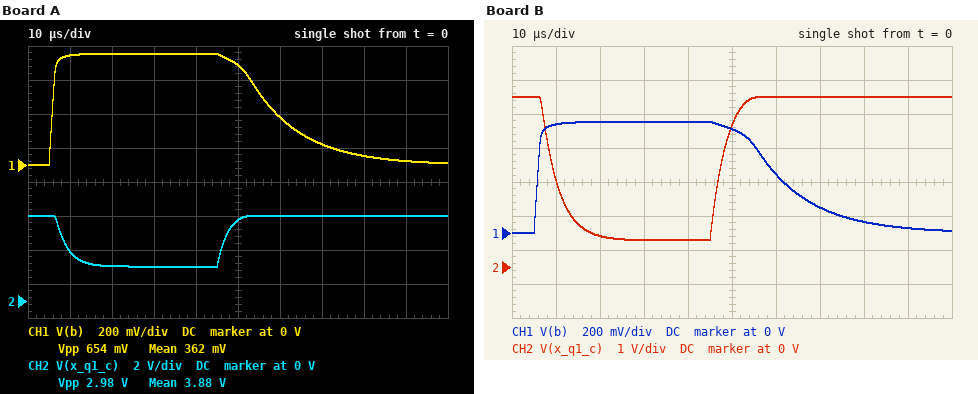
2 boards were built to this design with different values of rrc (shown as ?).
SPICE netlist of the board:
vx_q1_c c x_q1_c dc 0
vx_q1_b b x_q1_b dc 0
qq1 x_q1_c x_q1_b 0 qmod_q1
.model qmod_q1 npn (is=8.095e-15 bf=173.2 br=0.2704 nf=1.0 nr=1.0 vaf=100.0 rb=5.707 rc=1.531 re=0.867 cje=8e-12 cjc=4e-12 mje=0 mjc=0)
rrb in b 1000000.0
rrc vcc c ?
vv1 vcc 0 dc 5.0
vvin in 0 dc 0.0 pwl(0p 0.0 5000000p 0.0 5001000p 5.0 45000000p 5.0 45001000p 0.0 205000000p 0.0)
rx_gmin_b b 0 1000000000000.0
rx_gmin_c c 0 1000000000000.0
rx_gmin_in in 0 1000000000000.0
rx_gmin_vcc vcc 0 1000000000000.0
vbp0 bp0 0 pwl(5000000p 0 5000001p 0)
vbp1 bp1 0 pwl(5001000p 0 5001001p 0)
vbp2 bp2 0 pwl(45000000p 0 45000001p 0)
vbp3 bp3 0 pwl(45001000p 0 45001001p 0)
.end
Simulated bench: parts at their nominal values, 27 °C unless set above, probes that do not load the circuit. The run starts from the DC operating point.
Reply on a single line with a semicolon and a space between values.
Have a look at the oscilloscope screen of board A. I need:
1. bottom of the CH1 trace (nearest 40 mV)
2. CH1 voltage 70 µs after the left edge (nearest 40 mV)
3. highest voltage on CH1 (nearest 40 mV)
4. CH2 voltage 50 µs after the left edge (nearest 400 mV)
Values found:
0 V; 120 mV; 640 mV; 4.8 V
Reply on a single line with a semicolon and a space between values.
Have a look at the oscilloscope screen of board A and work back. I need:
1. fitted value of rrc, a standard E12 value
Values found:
3.9 kΩ
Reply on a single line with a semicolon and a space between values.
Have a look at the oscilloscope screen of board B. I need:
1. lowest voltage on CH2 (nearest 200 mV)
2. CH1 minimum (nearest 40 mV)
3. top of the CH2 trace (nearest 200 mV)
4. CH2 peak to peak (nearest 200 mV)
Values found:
800 mV; 0 V; 5.0 V; 4.2 V
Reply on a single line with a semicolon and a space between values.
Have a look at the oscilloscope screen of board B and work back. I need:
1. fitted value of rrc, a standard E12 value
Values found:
5.6 kΩ
